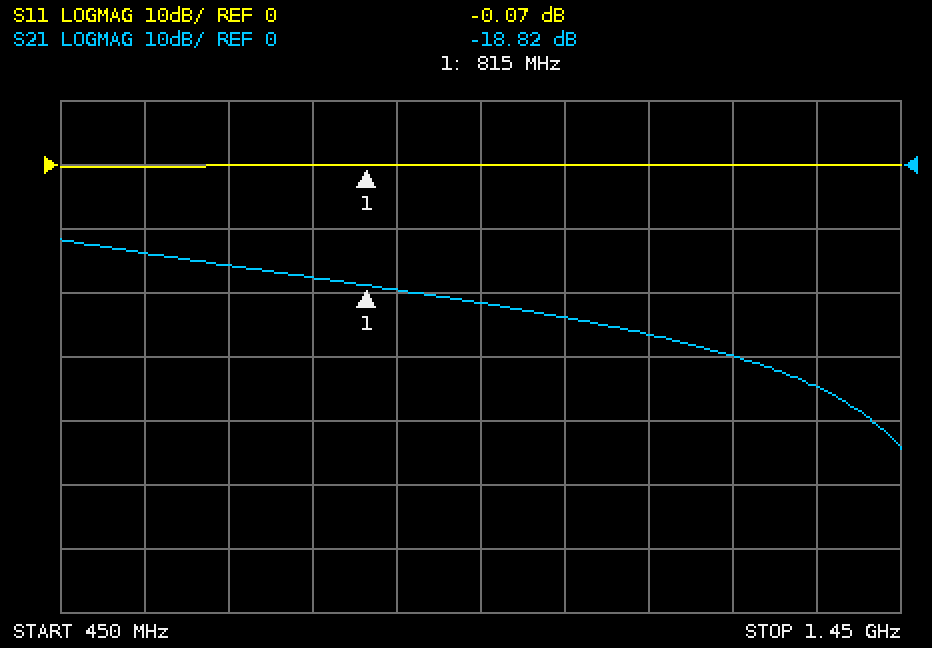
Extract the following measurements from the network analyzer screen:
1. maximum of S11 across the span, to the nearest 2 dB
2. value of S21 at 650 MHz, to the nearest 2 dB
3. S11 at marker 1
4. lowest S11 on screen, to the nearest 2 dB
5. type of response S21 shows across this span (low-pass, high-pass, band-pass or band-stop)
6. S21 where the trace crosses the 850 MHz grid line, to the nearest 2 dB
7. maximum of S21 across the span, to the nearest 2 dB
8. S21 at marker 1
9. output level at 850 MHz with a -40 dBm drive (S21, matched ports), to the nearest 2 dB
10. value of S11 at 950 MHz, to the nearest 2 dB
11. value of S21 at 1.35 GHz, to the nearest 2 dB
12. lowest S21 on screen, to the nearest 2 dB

0 dB
-16 dB
-0.07 dB
0 dB
low-pass
-20 dB
-12 dB
-18.82 dB
-60 dBm
0 dB
-34 dB
-44 dB
